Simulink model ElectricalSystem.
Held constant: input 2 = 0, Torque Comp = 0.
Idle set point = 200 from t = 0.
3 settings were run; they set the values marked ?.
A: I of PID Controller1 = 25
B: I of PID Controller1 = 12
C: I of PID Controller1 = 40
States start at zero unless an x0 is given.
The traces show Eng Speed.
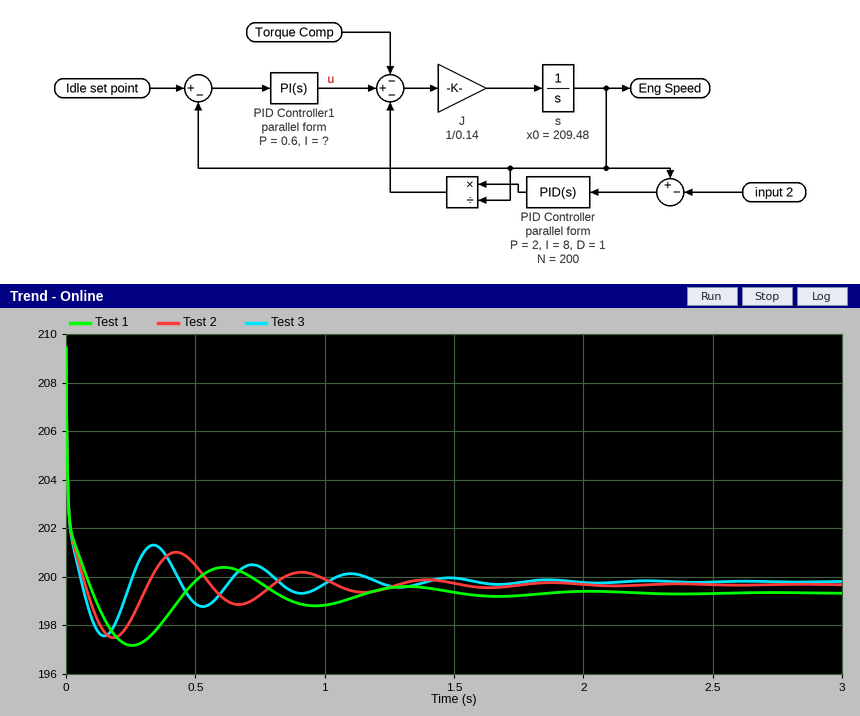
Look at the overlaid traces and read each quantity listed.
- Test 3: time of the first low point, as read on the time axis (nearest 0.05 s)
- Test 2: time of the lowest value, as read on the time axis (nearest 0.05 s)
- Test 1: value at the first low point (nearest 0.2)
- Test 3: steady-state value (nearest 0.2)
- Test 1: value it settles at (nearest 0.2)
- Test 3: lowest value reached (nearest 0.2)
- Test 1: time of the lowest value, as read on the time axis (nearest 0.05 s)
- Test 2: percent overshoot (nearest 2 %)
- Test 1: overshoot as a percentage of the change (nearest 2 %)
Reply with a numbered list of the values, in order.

1. 0.15 s
2. 0.20 s
3. 197.2
4. 199.8
5. 199.4
6. 197.6
7. 0.25 s
8. 22 %
9. 22 %
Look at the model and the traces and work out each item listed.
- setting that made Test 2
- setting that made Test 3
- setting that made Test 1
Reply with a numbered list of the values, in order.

1. A
2. C
3. B
